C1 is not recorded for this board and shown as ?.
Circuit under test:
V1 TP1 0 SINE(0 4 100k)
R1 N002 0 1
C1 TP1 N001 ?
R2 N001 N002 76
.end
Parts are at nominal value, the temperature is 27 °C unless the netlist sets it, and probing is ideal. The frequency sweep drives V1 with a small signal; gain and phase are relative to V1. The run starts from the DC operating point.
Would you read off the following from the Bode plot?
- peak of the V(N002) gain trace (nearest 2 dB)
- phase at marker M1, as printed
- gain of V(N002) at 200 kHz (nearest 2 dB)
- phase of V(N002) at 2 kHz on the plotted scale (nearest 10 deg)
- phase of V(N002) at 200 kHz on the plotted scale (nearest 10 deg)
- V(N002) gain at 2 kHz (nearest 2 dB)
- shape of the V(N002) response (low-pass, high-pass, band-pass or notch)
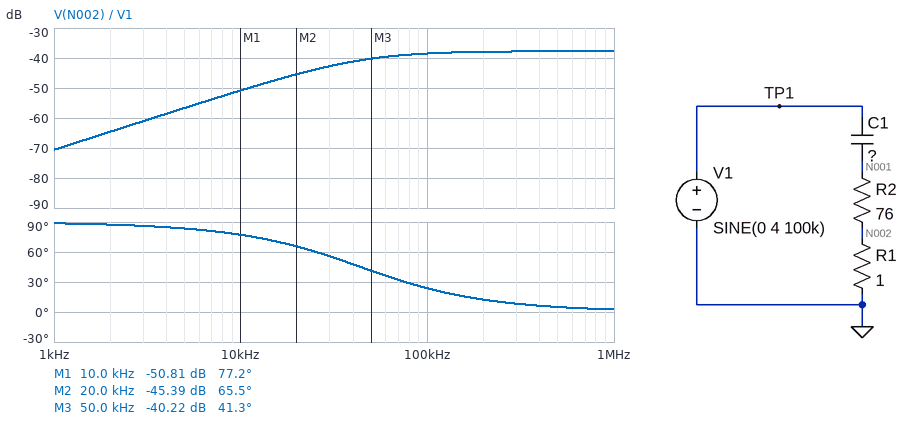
-38 dB
77.2 deg
-38 dB
90 deg
10 deg
-64 dB
high-pass
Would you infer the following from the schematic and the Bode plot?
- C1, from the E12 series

47 nF
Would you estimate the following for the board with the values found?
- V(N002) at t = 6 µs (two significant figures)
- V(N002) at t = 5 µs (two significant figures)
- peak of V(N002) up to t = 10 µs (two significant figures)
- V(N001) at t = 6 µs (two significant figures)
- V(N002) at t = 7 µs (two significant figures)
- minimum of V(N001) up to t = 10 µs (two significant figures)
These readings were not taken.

-45 mV
-24 mV
36 mV
-3.4 V
-50 mV
-3.9 V
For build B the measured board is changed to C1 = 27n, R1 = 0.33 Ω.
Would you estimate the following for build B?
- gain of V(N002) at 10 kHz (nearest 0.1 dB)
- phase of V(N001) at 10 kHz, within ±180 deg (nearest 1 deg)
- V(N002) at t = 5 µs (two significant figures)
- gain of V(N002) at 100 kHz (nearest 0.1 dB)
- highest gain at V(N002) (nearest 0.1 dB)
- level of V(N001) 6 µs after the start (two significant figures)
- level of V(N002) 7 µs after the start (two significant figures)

-65.1 dB
83 deg
-9.1 mV
-49.3 dB
-47.3 dB
-3.1 V
-13 mV
